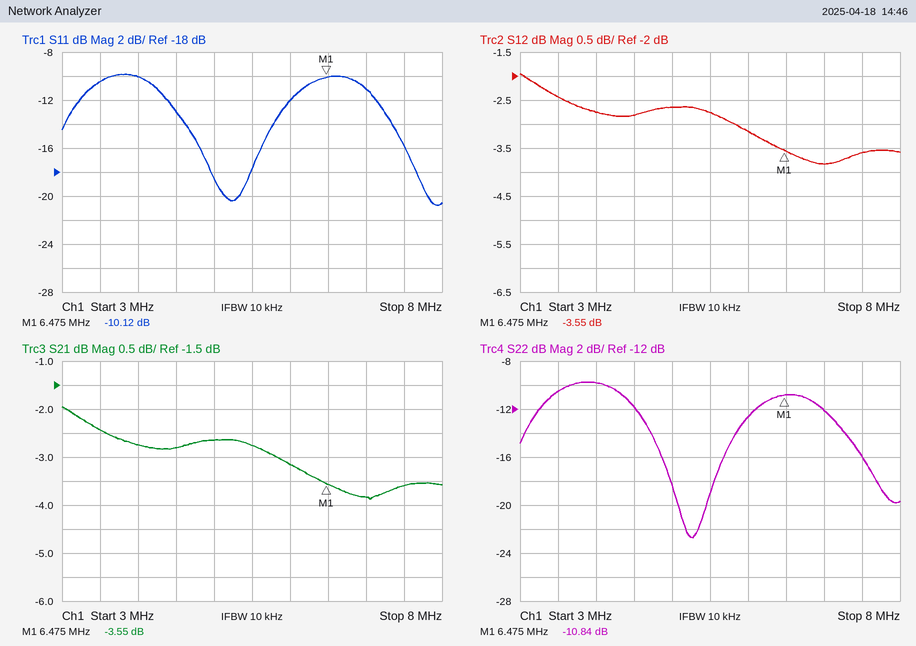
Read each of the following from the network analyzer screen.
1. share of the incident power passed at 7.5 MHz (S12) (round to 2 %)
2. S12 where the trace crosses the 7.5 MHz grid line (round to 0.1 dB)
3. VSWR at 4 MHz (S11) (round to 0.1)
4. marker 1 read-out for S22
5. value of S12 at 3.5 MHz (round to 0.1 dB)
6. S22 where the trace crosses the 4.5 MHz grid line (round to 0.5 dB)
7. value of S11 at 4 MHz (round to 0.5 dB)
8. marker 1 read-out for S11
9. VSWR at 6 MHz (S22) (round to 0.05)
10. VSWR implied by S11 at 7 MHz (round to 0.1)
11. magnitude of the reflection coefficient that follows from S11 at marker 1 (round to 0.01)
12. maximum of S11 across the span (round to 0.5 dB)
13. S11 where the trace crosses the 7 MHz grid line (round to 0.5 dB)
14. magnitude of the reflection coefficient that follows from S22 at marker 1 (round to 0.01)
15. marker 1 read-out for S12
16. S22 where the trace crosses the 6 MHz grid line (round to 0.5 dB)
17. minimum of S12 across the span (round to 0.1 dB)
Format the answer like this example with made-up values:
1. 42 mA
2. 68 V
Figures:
1. 44 %
2. -3.6 dB
3. 1.9
4. -10.84 dB
5. -2.4 dB
6. -12.0 dB
7. -10.0 dB
8. -10.12 dB
9. 1.60
10. 1.8
11. 0.31
12. -10.0 dB
13. -11.0 dB
14. 0.29
15. -3.55 dB
16. -12.5 dB
17. -3.8 dB
